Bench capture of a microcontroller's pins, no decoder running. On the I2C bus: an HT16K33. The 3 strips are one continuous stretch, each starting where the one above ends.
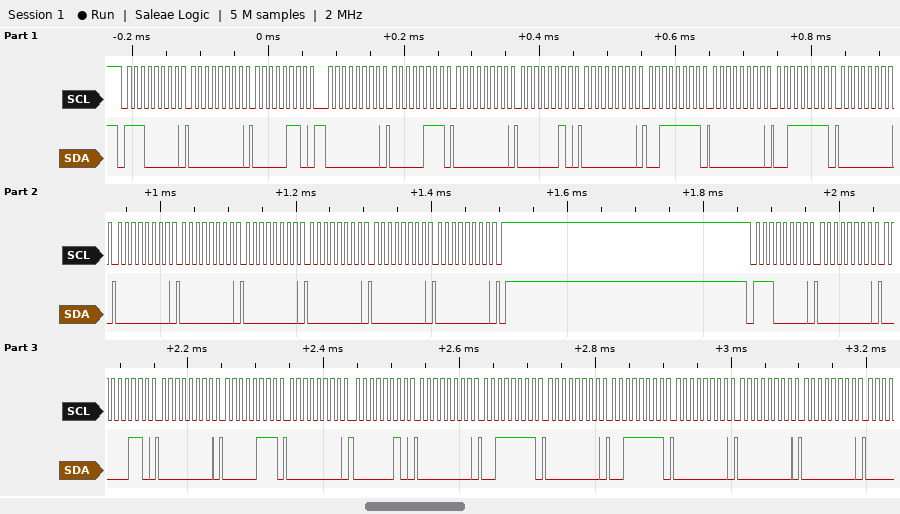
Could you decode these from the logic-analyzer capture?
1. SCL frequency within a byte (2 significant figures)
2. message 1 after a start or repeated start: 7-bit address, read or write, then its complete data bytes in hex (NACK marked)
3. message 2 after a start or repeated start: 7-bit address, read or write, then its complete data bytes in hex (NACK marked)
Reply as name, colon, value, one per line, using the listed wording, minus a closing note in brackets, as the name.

SCL frequency within a byte: 100 kHz
message 1 after a start or repeated start: 7-bit address, read or write, then its complete data bytes in hex: 0x70 write: 00 06 00 07 00 02 00 3F 00 3F 00 00 00 00 00 00 00
message 2 after a start or repeated start: 7-bit address, read or write, then its complete data bytes in hex: 0x70 write: 00 06 00 07 00 02 00 3F 00 3F 00 00 00
